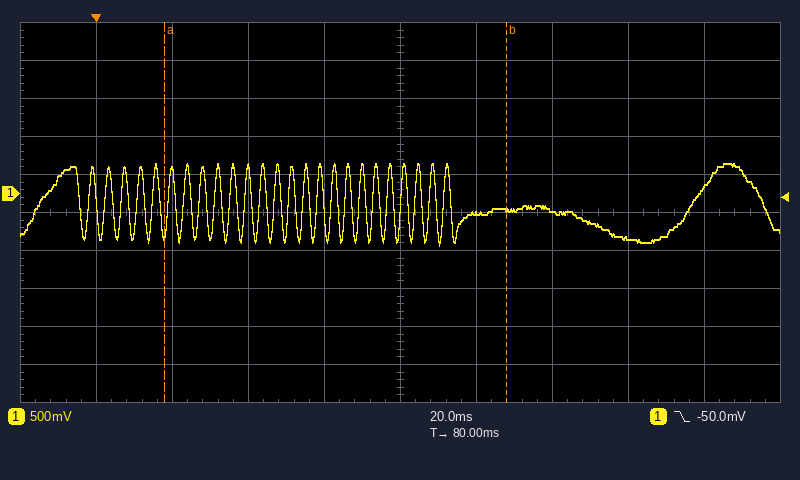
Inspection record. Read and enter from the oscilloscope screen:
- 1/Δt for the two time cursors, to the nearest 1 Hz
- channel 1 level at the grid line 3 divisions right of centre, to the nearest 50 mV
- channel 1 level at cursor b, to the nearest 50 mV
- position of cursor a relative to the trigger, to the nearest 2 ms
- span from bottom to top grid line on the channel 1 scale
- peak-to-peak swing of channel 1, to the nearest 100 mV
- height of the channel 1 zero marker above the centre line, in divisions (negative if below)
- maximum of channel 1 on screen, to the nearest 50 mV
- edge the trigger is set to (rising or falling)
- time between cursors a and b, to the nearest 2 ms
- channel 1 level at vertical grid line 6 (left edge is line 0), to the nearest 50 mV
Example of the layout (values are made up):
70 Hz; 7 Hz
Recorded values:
11 Hz; -600 mV; -200 mV; +18 ms; 5 V; 1.10 V; +0.5 div; 400 mV; falling; 90 ms; -250 mV
